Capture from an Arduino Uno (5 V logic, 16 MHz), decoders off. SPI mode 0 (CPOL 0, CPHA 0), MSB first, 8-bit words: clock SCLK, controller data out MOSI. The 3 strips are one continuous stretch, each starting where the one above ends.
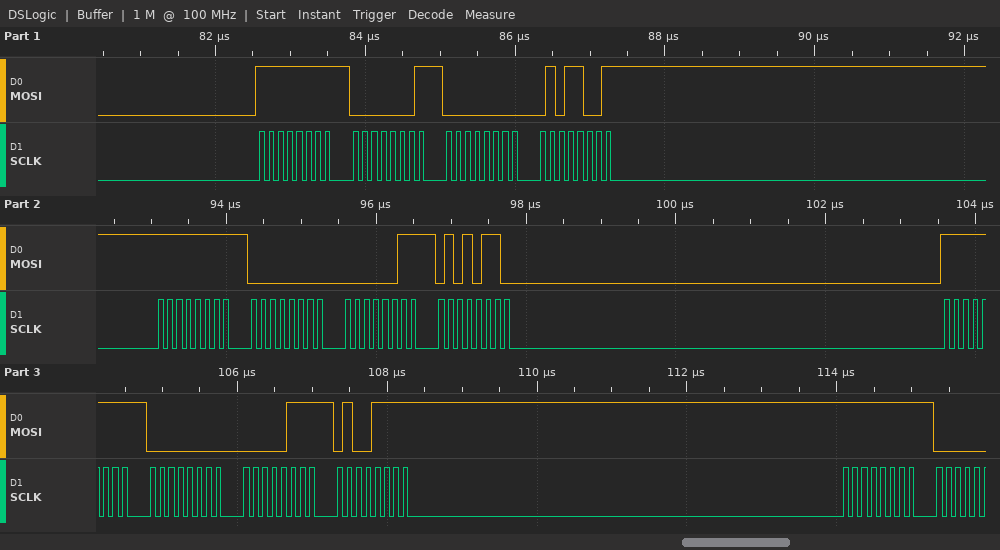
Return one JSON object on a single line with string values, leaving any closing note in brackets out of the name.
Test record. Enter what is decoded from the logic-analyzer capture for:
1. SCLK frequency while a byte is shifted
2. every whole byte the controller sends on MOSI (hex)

{"SCLK frequency while a byte is shifted": "8 MHz", "every whole byte the controller sends on MOSI": "FF 01 00 59 FF 00 03 56 FF 00 07 4F FF"}
